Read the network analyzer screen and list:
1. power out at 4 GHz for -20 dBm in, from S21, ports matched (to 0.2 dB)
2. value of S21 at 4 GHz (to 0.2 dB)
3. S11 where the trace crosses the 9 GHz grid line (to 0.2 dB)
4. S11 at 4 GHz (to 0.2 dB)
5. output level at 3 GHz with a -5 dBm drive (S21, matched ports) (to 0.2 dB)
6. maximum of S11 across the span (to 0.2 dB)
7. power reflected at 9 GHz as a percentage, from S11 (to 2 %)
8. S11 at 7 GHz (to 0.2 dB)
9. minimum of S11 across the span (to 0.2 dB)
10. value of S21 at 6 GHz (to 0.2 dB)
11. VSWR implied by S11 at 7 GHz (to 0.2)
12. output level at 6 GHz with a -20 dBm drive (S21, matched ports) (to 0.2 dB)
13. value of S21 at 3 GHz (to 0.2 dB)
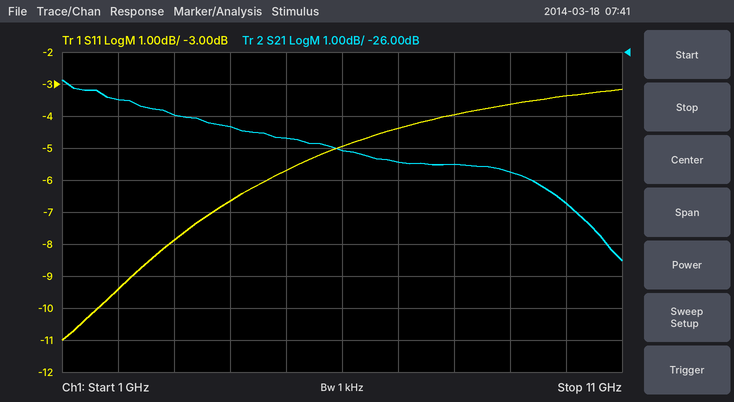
-48.4 dBm
-28.4 dB
-3.6 dB
-6.6 dB
-33.0 dBm
-3.2 dB
44 %
-4.4 dB
-11.0 dB
-29.0 dB
4.0
-49.0 dBm
-28.0 dB
